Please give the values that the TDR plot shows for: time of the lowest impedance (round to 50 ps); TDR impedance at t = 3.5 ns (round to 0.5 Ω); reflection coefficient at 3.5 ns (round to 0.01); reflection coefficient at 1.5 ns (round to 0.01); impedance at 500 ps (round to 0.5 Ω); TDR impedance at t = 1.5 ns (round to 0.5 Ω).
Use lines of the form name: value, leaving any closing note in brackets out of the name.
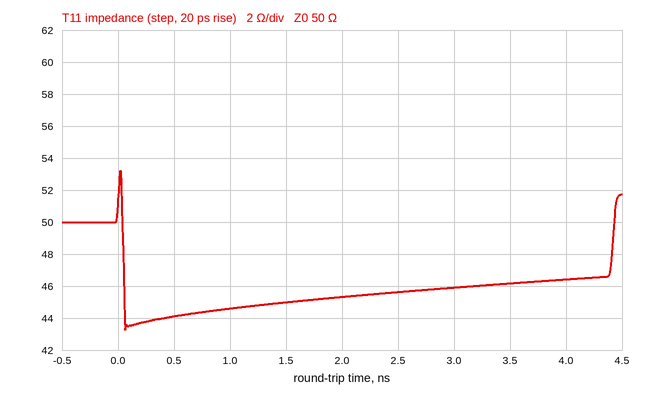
time of the lowest impedance: 50 ps
TDR impedance at t = 3.5 ns: 46.0 Ω
reflection coefficient at 3.5 ns: -0.04
reflection coefficient at 1.5 ns: -0.05
impedance at 500 ps: 44.0 Ω
TDR impedance at t = 1.5 ns: 45.0 Ω
